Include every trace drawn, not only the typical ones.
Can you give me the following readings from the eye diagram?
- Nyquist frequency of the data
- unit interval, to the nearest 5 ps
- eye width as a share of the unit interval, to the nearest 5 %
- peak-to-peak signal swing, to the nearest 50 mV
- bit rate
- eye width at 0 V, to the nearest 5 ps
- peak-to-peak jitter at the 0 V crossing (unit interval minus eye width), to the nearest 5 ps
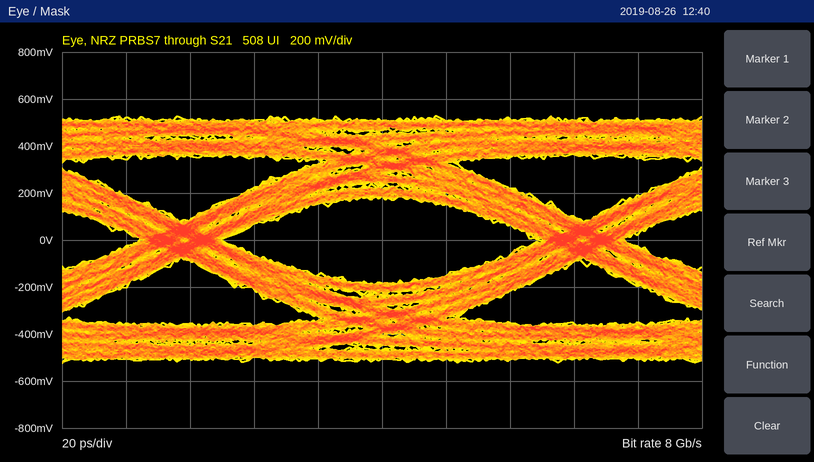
4 GHz
125 ps
80 %
1.05 V
8 Gb/s
100 ps
25 ps
